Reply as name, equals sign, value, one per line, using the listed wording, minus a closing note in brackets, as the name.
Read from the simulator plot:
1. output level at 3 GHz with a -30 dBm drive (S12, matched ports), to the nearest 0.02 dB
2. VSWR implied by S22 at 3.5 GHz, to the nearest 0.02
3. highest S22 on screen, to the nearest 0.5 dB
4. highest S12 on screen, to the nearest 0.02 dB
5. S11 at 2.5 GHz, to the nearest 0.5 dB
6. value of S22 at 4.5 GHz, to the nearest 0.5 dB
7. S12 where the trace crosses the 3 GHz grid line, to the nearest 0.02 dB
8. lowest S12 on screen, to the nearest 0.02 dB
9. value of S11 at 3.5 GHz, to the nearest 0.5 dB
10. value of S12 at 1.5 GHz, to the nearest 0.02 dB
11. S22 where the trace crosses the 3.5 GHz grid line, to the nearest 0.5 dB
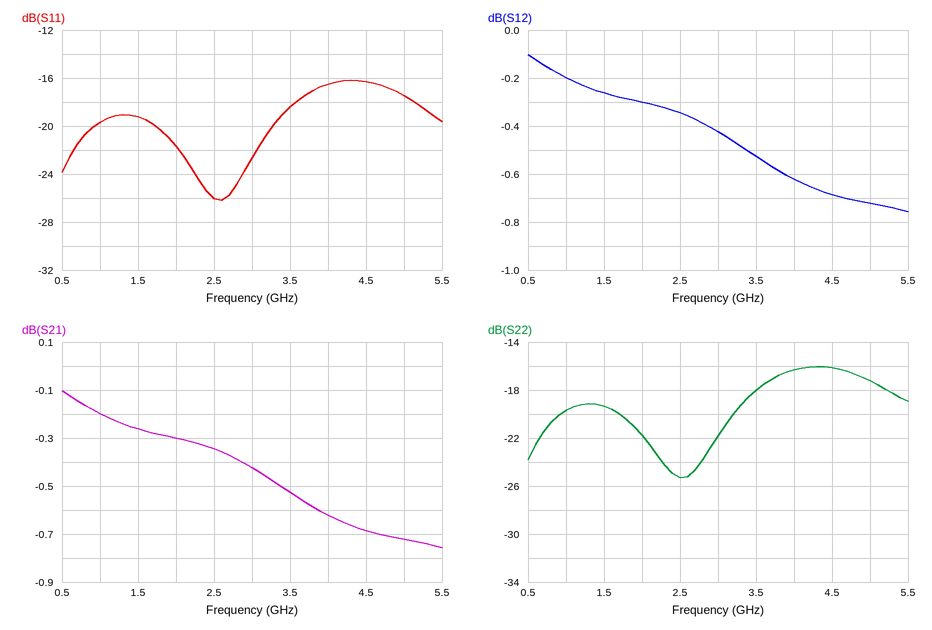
output level at 3 GHz with a -30 dBm drive (S12, matched ports), to the nearest 0.02 dB = -30.42 dBm
VSWR implied by S22 at 3.5 GHz, to the nearest 0.02 = 1.28
highest S22 on screen, to the nearest 0.5 dB = -16.0 dB
highest S12 on screen, to the nearest 0.02 dB = -0.10 dB
S11 at 2.5 GHz, to the nearest 0.5 dB = -26.0 dB
value of S22 at 4.5 GHz, to the nearest 0.5 dB = -16.0 dB
S12 where the trace crosses the 3 GHz grid line, to the nearest 0.02 dB = -0.42 dB
lowest S12 on screen, to the nearest 0.02 dB = -0.76 dB
value of S11 at 3.5 GHz, to the nearest 0.5 dB = -18.5 dB
value of S12 at 1.5 GHz, to the nearest 0.02 dB = -0.26 dB
S22 where the trace crosses the 3.5 GHz grid line, to the nearest 0.5 dB = -18.0 dB
